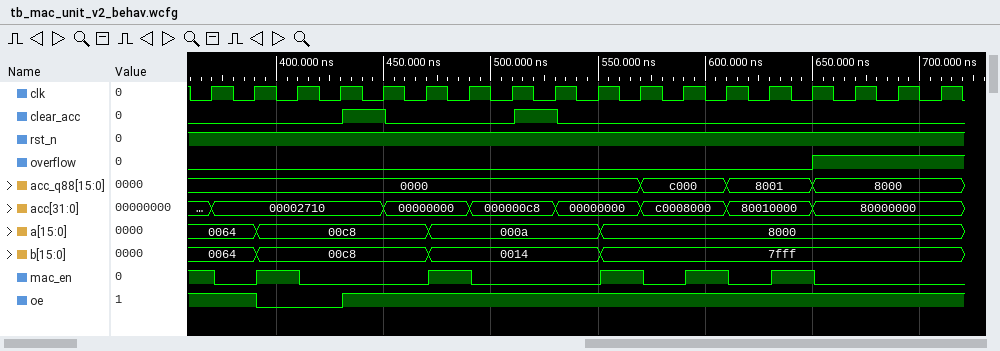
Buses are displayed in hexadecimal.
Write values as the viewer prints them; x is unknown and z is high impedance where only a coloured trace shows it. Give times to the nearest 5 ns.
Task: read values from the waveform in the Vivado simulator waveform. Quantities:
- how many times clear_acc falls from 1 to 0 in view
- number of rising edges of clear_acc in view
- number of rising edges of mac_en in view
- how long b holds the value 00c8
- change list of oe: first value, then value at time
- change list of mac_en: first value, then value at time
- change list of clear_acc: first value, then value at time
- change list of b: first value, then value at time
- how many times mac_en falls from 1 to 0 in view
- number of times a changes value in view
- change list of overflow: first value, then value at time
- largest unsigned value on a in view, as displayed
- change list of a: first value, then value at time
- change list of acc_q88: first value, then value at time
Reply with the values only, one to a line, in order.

2
2
5
80 ns
1, 0 at 390 ns, 1 at 430 ns
1, 0 at 370 ns, 1 at 390 ns, 0 at 410 ns, 1 at 470 ns, 0 at 490 ns, 1 at 550 ns, 0 at 570 ns, 1 at 590 ns, 0 at 610 ns, 1 at 630 ns, 0 at 650 ns
0, 1 at 430 ns, 0 at 450 ns, 1 at 510 ns, 0 at 530 ns
0064, 00c8 at 390 ns, 0014 at 470 ns, 7fff at 550 ns
6
3
0, 1 at 650 ns
8000
0064, 00c8 at 390 ns, 000a at 470 ns, 8000 at 550 ns
0000, c000 at 570 ns, 8001 at 610 ns, 8000 at 650 ns
